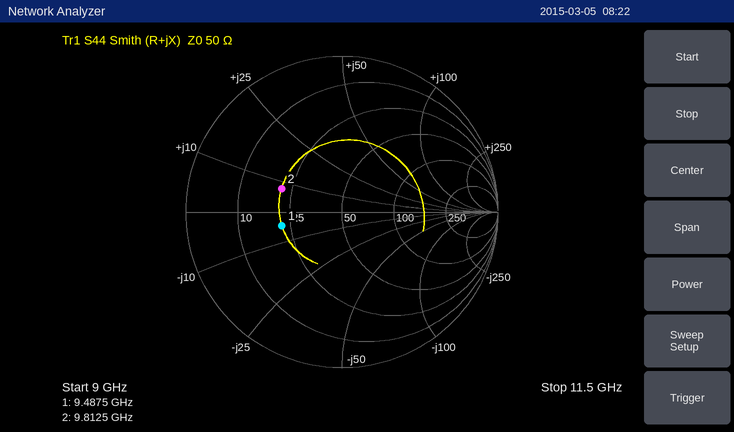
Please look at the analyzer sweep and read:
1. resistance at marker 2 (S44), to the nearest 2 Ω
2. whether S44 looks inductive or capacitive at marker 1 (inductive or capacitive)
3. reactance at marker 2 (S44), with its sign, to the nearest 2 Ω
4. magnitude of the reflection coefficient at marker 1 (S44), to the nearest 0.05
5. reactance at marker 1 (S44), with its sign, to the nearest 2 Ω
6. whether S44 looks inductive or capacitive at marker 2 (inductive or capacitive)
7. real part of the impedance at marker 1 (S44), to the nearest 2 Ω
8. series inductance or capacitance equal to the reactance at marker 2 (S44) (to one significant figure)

22 Ω
capacitive
+8 Ω
0.40
-4 Ω
inductive
22 Ω
100 pH
